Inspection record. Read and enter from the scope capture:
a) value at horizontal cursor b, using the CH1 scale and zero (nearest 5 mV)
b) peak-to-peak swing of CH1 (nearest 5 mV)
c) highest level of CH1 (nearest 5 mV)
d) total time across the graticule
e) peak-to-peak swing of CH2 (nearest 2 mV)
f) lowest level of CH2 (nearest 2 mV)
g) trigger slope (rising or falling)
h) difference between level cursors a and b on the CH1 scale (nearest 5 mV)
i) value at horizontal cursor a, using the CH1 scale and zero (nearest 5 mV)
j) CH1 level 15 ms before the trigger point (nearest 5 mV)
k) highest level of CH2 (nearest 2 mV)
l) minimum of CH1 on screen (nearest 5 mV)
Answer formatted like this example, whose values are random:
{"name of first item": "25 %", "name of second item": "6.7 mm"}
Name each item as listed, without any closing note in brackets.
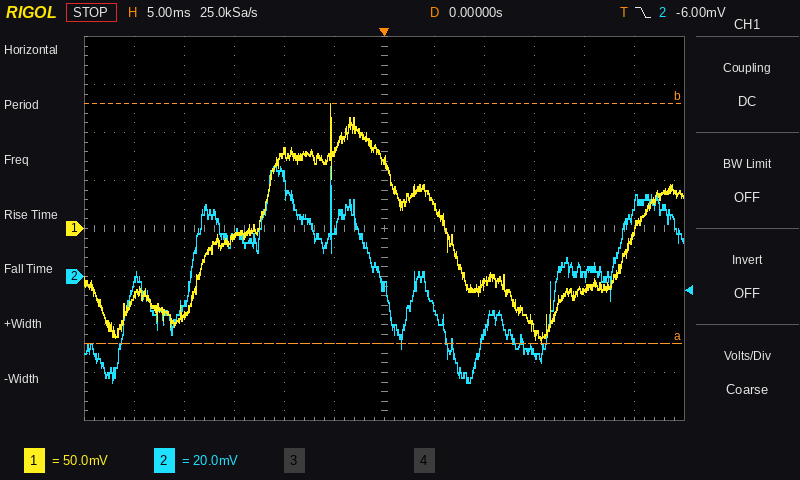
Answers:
{"value at horizontal cursor b, using the CH1 scale and zero": "130 mV", "peak-to-peak swing of CH1": "250 mV", "highest level of CH1": "130 mV", "total time across the graticule": "60 ms", "peak-to-peak swing of CH2": "90 mV", "lowest level of CH2": "-44 mV", "trigger slope": "falling", "difference between level cursors a and b on the CH1 scale": "250 mV", "value at horizontal cursor a, using the CH1 scale and zero": "-120 mV", "CH1 level 15 ms before the trigger point": "-10 mV", "highest level of CH2": "46 mV", "minimum of CH1 on screen": "-120 mV"}
